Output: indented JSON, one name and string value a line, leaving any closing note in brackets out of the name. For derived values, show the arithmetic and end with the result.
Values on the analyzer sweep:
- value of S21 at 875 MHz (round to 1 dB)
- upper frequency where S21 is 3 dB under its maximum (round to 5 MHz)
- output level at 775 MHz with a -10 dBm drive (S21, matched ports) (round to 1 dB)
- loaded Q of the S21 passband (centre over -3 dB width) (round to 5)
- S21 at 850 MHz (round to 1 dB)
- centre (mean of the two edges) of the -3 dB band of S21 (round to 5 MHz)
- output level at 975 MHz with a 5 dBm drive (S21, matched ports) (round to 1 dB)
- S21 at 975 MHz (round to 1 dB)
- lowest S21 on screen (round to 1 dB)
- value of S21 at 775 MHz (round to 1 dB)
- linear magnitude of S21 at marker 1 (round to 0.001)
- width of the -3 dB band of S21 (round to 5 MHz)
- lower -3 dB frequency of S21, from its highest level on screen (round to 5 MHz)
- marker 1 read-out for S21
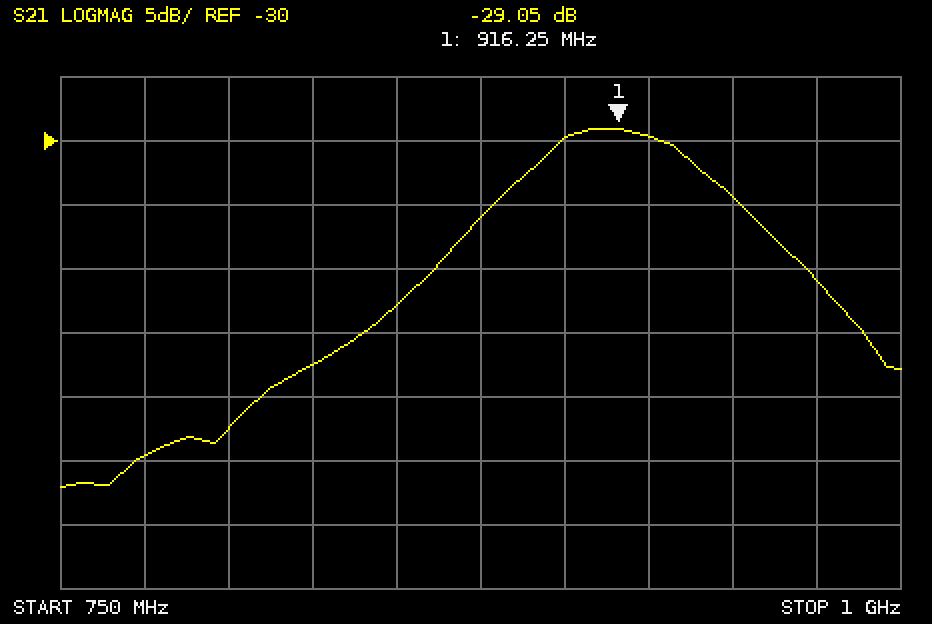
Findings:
{
  "value of S21 at 875 MHz": "-36 dB",
  "upper frequency where S21 is 3 dB under its maximum": "940 MHz",
  "output level at 775 MHz with a -10 dBm drive (S21, matched ports)": "-10 dBm + (-55 dB) = -65 dBm",
  "loaded Q of the S21 passband (centre over -3 dB width)": "915 MHz / 50 MHz ≈ 18.3, so 20 to the nearest 5",
  "S21 at 850 MHz": "-43 dB",
  "centre (mean of the two edges) of the -3 dB band of S21": "915 MHz",
  "output level at 975 MHz with a 5 dBm drive (S21, matched ports)": "5 dBm + (-41 dB) = -36 dBm",
  "S21 at 975 MHz": "-41 dB",
  "lowest S21 on screen": "-57 dB",
  "value of S21 at 775 MHz": "-55 dB",
  "linear magnitude of S21 at marker 1": "10^(-29.05/20) ≈ 0.035",
  "width of the -3 dB band of S21": "940 MHz − 890 MHz = 50 MHz",
  "lower -3 dB frequency of S21, from its highest level on screen": "890 MHz",
  "marker 1 read-out for S21": "-29.05 dB"
}
